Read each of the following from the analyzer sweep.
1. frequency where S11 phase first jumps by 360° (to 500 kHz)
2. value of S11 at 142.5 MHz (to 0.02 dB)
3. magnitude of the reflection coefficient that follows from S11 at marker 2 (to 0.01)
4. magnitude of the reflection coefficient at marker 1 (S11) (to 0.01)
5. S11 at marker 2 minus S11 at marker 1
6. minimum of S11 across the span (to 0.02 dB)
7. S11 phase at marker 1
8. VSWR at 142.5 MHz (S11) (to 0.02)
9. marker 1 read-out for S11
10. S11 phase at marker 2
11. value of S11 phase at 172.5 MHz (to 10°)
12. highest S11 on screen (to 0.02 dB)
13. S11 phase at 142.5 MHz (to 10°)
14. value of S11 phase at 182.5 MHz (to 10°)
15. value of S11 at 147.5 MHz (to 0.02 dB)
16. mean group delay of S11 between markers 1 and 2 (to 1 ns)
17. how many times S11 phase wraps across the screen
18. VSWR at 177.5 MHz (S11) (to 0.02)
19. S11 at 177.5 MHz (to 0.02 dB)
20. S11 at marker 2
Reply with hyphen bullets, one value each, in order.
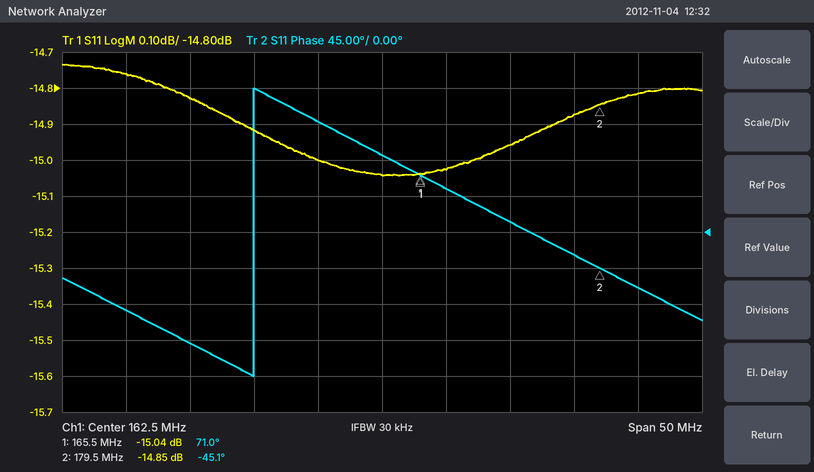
- 152.5 MHz
- -14.76 dB
- 0.18
- 0.18
- 0.19 dB
- -15.04 dB
- 71.0°
- 1.44
- -15.04 dB
- -45.1°
- 10°
- -14.74 dB
- -100°
- -70°
- -14.82 dB
- 23 ns
- 1
- 1.44
- -14.88 dB
- -14.85 dB
